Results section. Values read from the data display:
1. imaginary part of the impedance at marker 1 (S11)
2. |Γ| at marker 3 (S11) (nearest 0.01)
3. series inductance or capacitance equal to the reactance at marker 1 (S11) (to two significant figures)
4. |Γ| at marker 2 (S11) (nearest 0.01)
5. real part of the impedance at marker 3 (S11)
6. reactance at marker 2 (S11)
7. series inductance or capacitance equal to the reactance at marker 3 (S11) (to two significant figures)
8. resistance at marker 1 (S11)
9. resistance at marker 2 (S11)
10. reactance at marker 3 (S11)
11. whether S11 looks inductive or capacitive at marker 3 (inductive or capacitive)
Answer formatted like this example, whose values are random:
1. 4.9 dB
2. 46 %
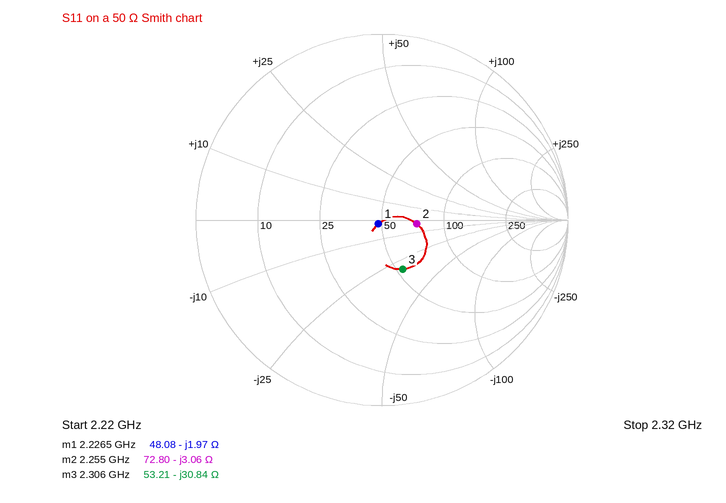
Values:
1. -1.97 Ω
2. 0.29
3. 36 pF
4. 0.19
5. 53.21 Ω
6. -3.06 Ω
7. 2.2 pF
8. 48.08 Ω
9. 72.80 Ω
10. -30.84 Ω
11. capacitive
